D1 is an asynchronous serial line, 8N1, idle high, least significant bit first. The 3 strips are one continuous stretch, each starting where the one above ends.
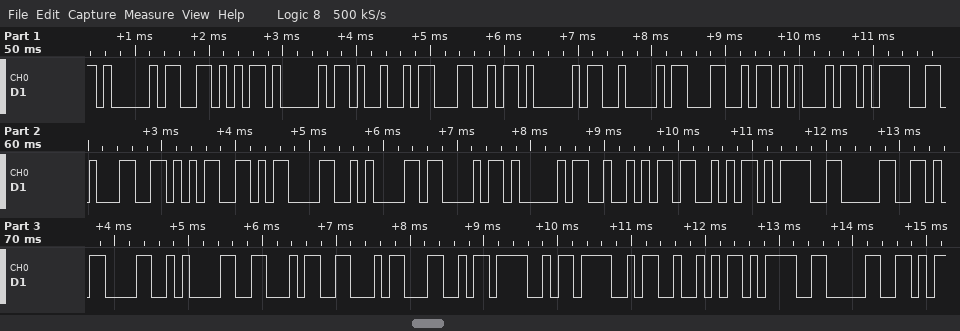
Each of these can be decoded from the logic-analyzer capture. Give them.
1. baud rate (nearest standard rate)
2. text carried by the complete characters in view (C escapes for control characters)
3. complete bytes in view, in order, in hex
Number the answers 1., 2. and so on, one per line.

1. 9600 baud
2. "AVAILABLE=15\r\nCARS=0\r\nFFLOOR=0"
3. 41 56 41 49 4C 41 42 4C 45 3D 31 35 0D 0A 43 41 52 53 3D 30 0D 0A 46 46 4C 4F 4F 52 3D 30
